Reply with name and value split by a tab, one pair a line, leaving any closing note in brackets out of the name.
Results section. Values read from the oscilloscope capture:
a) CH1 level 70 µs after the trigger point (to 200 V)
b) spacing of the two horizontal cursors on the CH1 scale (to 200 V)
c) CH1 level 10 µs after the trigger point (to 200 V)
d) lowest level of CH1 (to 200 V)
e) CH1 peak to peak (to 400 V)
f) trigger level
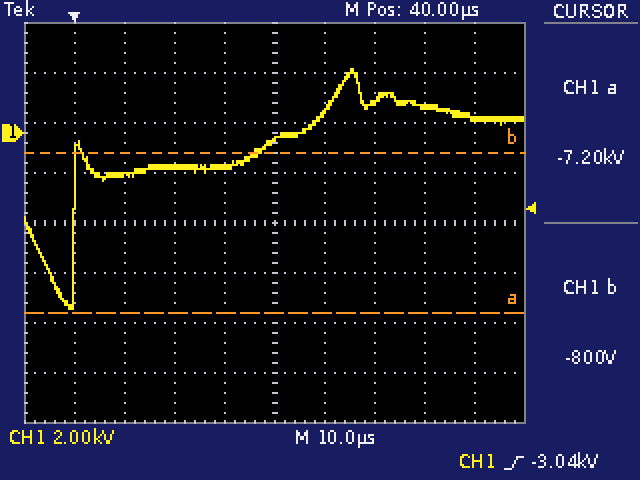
CH1 level 70 µs after the trigger point	1.0 kV
spacing of the two horizontal cursors on the CH1 scale	6.4 kV
CH1 level 10 µs after the trigger point	-1.6 kV
lowest level of CH1	-7.0 kV
CH1 peak to peak	9.6 kV
trigger level	-3.04 kV
